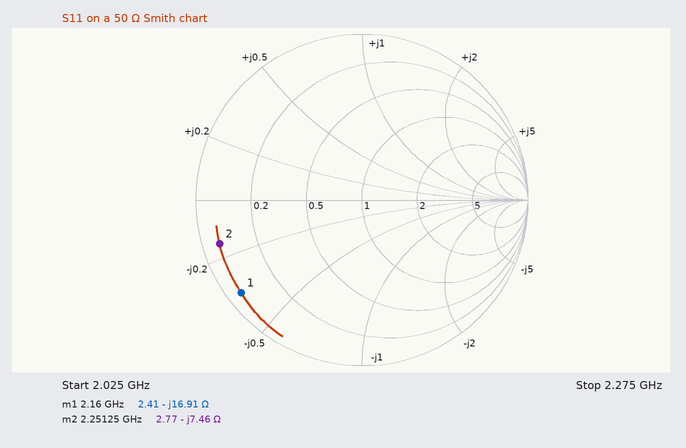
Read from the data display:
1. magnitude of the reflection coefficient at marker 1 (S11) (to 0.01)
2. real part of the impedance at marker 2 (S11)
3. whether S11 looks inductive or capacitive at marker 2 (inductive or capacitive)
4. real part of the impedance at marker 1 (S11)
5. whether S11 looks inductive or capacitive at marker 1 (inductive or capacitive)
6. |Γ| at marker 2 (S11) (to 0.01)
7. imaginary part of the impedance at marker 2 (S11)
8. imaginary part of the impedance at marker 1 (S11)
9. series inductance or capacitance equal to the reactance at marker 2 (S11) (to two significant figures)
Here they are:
0.92
2.77 Ω
capacitive
2.41 Ω
capacitive
0.90
-7.46 Ω
-16.91 Ω
9.5 pF
